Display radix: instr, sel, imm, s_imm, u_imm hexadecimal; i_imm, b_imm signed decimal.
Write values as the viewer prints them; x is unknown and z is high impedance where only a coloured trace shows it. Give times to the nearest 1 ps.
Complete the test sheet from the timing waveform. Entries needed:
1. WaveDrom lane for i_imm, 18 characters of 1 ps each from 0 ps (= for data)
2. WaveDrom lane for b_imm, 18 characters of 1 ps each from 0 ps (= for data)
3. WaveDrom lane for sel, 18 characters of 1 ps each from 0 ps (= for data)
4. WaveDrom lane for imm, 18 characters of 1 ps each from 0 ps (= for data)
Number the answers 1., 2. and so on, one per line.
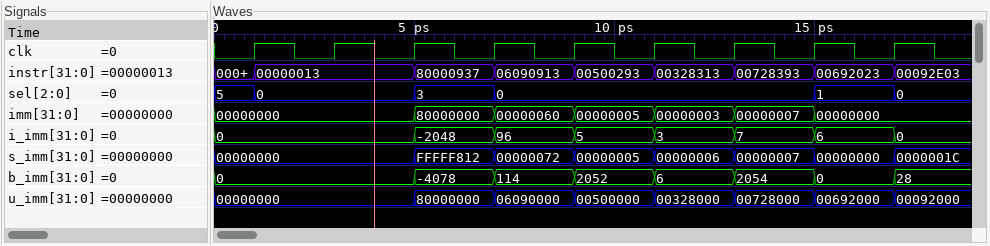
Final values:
1. {name: 'i_imm', wave: '=....=.=.=.=.=.=.=', data: '0 -2048 96 5 3 7 6 0'}
2. {name: 'b_imm', wave: '=....=.=.=.=.=.=.=', data: '0 -4078 114 2052 6 2054 0 28'}
3. {name: 'sel', wave: '==...=.=.......=.=', data: '5 0 3 0 1 0'}
4. {name: 'imm', wave: '=....=.=.=.=.=.=..', data: '00000000 80000000 00000060 00000005 00000003 00000007 00000000'}
